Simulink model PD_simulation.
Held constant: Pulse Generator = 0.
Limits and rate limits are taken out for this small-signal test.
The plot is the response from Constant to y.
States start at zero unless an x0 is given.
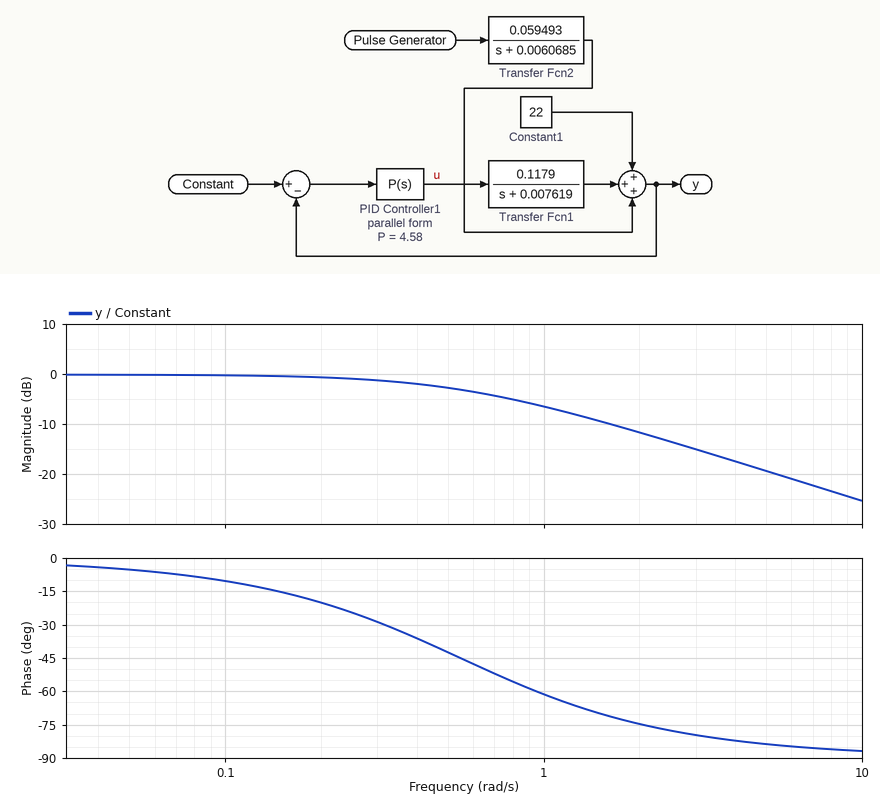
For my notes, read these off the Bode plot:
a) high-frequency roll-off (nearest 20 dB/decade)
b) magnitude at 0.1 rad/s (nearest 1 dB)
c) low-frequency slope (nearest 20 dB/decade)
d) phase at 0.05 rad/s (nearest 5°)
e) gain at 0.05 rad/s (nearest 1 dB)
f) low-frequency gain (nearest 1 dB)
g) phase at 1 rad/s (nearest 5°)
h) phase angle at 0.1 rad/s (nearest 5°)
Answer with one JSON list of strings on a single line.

["-20 dB/decade", "0 dB", "0 dB/decade", "-5°", "0 dB", "0 dB", "-60°", "-10°"]
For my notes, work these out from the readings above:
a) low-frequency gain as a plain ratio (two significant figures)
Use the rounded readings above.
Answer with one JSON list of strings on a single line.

["1.0"]
